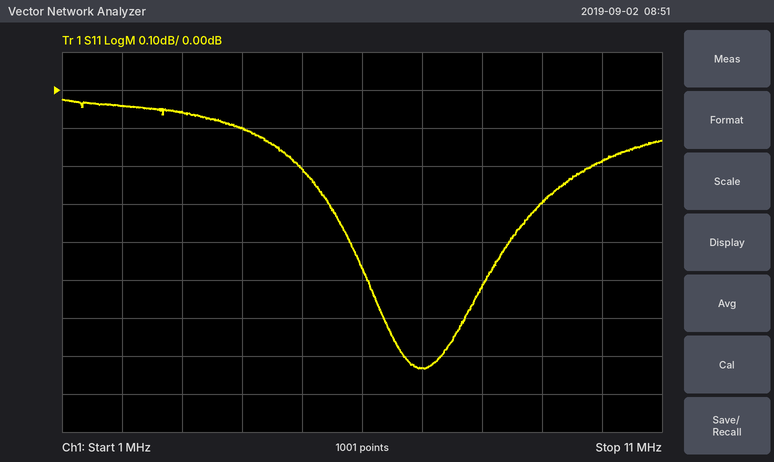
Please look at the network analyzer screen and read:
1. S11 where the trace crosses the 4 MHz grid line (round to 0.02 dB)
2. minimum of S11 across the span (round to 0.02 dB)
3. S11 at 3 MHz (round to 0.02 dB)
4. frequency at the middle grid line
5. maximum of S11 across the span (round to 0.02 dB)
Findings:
-0.10 dB
-0.74 dB
-0.06 dB
6 MHz
-0.02 dB
